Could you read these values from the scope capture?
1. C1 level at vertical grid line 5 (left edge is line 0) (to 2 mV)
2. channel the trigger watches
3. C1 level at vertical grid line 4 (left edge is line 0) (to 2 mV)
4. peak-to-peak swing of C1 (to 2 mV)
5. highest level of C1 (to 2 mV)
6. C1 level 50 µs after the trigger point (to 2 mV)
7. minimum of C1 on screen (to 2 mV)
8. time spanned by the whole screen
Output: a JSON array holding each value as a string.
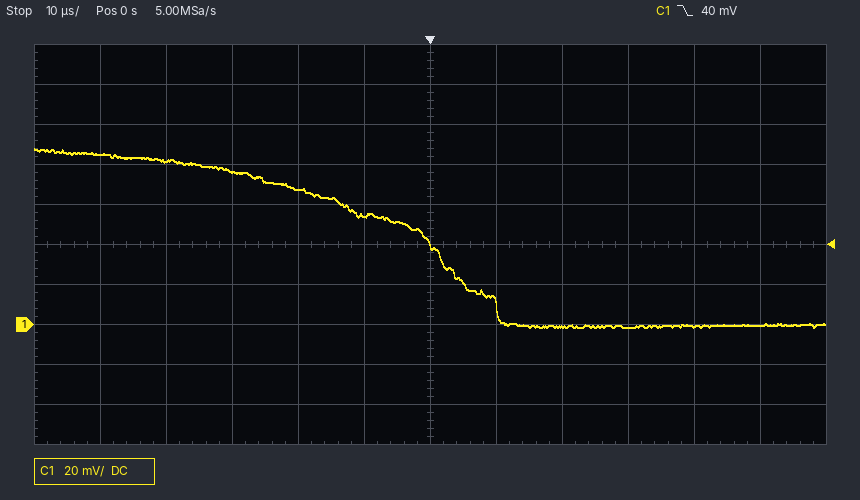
["54 mV", "C1", "68 mV", "90 mV", "88 mV", "0 mV", "-2 mV", "120 µs"]
